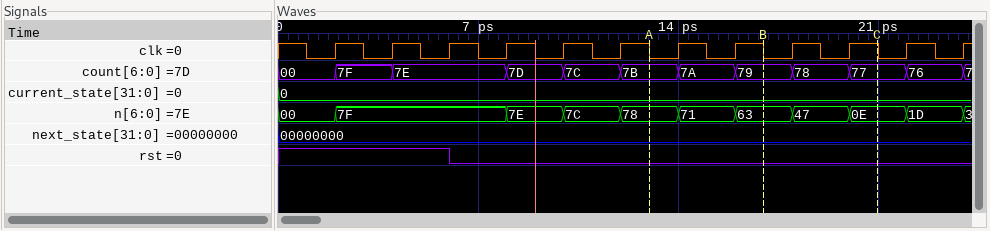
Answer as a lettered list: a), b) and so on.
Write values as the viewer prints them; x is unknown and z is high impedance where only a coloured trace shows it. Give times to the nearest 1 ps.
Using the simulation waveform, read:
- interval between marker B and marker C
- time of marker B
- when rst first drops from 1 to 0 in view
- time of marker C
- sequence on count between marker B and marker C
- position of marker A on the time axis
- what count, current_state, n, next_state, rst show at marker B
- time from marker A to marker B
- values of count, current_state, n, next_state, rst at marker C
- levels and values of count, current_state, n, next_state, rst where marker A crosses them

a) 4 ps
b) 17 ps
c) 6 ps
d) 21 ps
e) 79, 78, 77
f) 13 ps
g) count=79, current_state=0, n=63, next_state=00000000, rst=0
h) 4 ps
i) count=77, current_state=0, n=0E, next_state=00000000, rst=0
j) count=7B, current_state=0, n=78, next_state=00000000, rst=0
